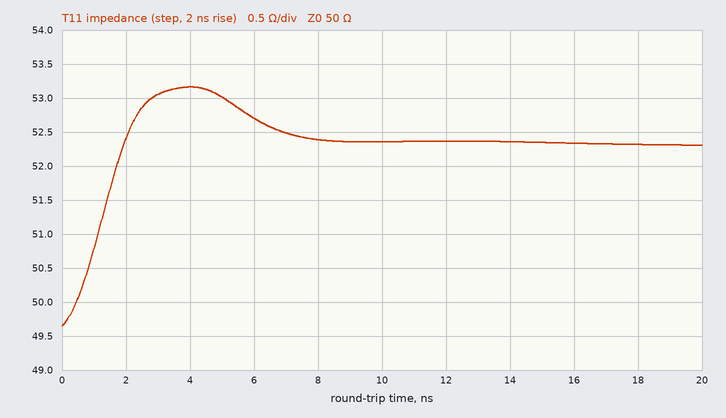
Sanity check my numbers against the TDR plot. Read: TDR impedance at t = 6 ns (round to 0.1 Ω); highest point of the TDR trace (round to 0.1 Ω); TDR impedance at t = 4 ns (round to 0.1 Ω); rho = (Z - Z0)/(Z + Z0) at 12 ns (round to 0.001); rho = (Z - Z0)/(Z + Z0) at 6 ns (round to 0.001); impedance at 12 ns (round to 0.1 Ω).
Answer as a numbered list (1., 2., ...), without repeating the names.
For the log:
1. 52.7 Ω
2. 53.2 Ω
3. 53.2 Ω
4. +0.023
5. +0.026
6. 52.4 Ω
